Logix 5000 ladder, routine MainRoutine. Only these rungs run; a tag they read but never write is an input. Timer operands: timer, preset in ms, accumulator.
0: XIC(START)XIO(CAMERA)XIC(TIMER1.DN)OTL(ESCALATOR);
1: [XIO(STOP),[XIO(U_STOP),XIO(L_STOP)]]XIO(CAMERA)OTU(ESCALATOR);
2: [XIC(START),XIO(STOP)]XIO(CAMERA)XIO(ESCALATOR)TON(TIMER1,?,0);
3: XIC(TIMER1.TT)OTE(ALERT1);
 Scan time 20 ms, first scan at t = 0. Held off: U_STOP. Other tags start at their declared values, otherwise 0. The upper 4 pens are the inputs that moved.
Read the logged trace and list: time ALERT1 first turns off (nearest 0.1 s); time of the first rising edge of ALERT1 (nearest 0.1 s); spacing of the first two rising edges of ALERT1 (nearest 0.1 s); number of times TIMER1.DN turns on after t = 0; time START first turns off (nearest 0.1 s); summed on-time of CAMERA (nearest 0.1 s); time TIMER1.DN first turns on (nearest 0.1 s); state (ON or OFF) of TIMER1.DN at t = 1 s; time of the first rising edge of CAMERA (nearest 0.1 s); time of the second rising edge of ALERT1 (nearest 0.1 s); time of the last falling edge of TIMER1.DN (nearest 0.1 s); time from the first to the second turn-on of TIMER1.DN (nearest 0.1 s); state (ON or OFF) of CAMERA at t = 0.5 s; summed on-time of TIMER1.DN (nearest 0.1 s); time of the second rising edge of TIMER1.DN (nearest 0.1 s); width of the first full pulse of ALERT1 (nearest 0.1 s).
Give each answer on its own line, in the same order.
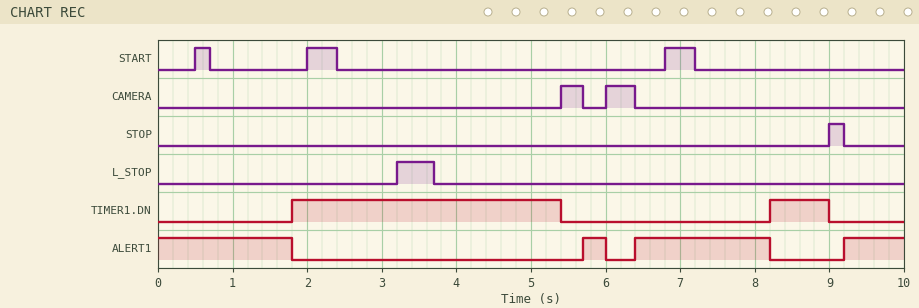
1.8 s
5.7 s
0.7 s
2
0.7 s
0.7 s
1.8 s
OFF
5.4 s
6.4 s
9.0 s
6.4 s
OFF
4.4 s
8.2 s
0.3 s
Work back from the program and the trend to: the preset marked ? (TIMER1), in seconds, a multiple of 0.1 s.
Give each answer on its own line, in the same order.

1.8 s
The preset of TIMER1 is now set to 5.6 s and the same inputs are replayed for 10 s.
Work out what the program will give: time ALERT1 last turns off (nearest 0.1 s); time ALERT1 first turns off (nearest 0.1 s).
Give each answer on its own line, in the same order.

9.0 s
5.4 s
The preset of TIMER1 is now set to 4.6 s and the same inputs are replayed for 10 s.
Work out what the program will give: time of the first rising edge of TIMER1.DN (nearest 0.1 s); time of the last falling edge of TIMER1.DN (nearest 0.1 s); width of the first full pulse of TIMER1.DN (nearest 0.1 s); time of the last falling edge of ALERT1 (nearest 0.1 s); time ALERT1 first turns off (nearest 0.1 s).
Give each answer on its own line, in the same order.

4.6 s
5.4 s
0.8 s
9.0 s
4.6 s
